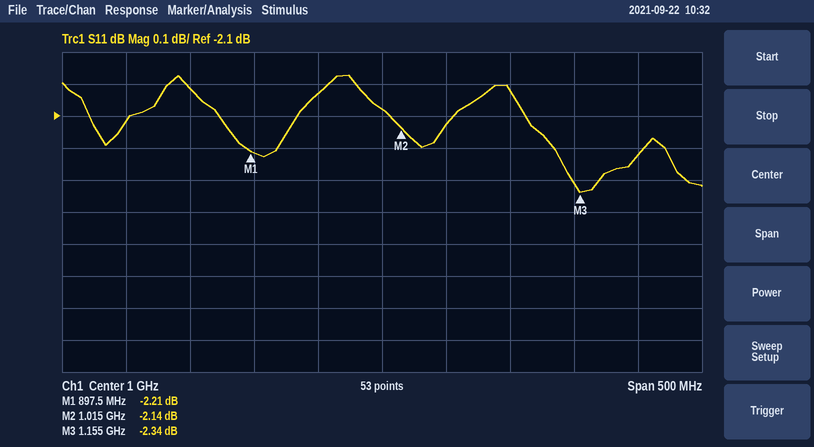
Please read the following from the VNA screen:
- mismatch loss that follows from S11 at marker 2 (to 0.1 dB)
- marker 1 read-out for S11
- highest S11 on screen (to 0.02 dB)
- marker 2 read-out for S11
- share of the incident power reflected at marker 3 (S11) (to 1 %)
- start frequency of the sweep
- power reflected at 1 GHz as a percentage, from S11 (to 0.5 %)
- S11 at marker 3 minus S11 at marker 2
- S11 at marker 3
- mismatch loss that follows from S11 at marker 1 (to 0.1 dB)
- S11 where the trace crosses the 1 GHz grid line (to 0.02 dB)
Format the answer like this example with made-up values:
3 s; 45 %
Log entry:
4.1 dB; -2.21 dB; -1.98 dB; -2.14 dB; 58 %; 750 MHz; 62.0 %; -0.20 dB; -2.34 dB; 4.0 dB; -2.08 dB
